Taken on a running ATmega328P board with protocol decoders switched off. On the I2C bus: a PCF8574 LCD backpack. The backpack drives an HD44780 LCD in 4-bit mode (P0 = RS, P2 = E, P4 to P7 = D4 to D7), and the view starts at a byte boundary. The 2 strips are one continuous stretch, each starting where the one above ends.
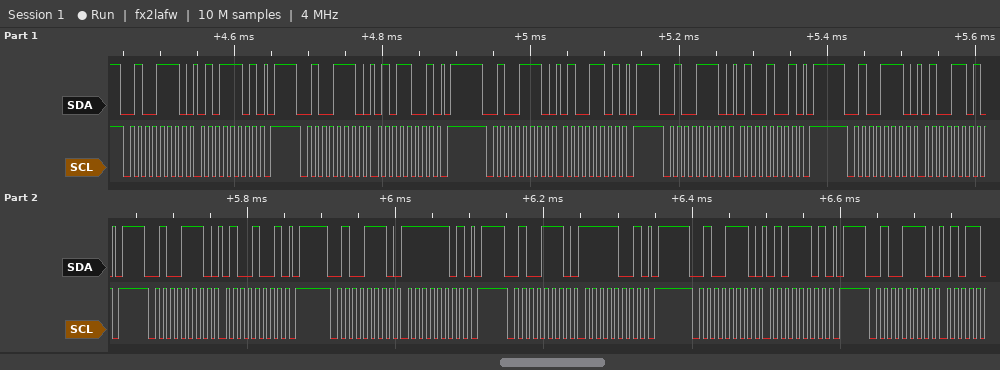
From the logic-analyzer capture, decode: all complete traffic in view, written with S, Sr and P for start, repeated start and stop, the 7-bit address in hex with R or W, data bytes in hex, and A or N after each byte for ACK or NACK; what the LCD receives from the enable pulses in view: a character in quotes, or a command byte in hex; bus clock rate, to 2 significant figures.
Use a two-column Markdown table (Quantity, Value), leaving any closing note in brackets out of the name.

| Quantity | Value |
|---|---|
| all complete traffic in view, written with S, Sr and P for start, repeated start and stop, the 7-bit address in hex with R or W, data bytes in hex, and A or N after each byte for ACK or NACK | S 27W A 5D A P S 27W A 59 A P S 27W A 4D A P S 27W A 49 A P S 27W A 4D A P S 27W A 49 A P S 27W A FD A P S 27W A F9 A P S 27W A 5D A P S 27W A |
| what the LCD receives from the enable pulses in view: a character in quotes, or a command byte in hex | 'T' 'O' |
| bus clock rate, to 2 significant figures | 100 kHz |
